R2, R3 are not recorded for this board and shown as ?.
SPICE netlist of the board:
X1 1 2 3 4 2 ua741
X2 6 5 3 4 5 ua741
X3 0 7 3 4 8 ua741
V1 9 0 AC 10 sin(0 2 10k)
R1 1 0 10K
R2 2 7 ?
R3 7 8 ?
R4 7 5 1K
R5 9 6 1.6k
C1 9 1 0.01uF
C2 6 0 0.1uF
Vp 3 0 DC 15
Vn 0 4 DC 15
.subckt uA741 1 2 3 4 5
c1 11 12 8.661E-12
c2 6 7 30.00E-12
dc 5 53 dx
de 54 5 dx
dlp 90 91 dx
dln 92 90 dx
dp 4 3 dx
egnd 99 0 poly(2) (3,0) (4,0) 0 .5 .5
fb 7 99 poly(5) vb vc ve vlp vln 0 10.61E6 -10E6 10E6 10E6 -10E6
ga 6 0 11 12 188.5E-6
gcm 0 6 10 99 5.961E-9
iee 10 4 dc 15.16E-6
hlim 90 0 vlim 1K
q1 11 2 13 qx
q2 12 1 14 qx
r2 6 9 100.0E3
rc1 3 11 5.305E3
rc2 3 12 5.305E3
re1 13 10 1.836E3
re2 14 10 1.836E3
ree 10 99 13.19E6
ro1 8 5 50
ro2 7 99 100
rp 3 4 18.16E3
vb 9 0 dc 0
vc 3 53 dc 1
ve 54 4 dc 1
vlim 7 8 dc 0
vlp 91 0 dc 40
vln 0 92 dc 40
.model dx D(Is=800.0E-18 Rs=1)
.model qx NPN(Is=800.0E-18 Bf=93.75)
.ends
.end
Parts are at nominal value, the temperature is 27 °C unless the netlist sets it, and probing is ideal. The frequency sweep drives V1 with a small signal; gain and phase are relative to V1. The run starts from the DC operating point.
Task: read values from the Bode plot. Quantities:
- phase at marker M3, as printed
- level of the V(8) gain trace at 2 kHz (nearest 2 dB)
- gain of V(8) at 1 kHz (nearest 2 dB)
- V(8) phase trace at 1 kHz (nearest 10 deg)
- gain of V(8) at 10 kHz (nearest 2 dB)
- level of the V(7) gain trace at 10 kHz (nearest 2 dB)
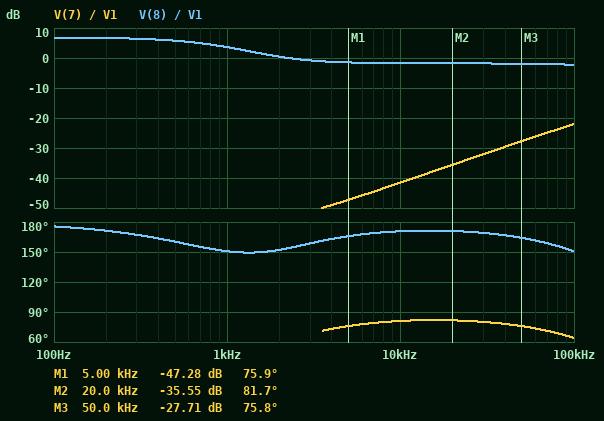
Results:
75.8 deg
0 dB
4 dB
150 deg
-2 dB
-42 dB
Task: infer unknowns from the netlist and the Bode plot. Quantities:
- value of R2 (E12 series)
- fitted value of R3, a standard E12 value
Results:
2.7 kΩ
2.2 kΩ
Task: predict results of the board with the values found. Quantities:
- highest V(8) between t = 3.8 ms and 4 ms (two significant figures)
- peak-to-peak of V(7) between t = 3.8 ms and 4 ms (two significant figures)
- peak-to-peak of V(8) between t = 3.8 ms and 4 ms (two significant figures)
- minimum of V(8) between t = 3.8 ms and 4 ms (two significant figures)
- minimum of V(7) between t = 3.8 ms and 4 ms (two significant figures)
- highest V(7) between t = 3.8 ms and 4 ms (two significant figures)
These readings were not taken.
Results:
1.6 V
34 mV
3.3 V
-1.6 V
-17 mV
17 mV
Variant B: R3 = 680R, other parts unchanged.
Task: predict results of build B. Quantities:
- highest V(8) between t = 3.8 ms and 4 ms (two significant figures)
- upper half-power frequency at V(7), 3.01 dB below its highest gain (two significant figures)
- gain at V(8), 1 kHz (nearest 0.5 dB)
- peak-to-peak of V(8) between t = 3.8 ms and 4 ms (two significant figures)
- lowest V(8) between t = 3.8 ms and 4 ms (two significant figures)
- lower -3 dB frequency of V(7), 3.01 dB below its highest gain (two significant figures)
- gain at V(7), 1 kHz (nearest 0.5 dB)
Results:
510 mV
1.5 MHz
-6.5 dB
1.0 V
-510 mV
420 kHz
-66.0 dB
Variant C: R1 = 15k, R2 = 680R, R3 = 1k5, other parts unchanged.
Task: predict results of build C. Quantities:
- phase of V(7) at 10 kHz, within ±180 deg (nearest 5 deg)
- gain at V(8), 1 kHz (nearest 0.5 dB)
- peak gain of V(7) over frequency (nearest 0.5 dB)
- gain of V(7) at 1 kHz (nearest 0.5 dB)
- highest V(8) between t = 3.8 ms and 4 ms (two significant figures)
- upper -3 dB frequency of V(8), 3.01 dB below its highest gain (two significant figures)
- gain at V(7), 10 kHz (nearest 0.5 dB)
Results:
90 deg
5.0 dB
-6.0 dB
-54.5 dB
4.4 V
230 kHz
-33.0 dB
